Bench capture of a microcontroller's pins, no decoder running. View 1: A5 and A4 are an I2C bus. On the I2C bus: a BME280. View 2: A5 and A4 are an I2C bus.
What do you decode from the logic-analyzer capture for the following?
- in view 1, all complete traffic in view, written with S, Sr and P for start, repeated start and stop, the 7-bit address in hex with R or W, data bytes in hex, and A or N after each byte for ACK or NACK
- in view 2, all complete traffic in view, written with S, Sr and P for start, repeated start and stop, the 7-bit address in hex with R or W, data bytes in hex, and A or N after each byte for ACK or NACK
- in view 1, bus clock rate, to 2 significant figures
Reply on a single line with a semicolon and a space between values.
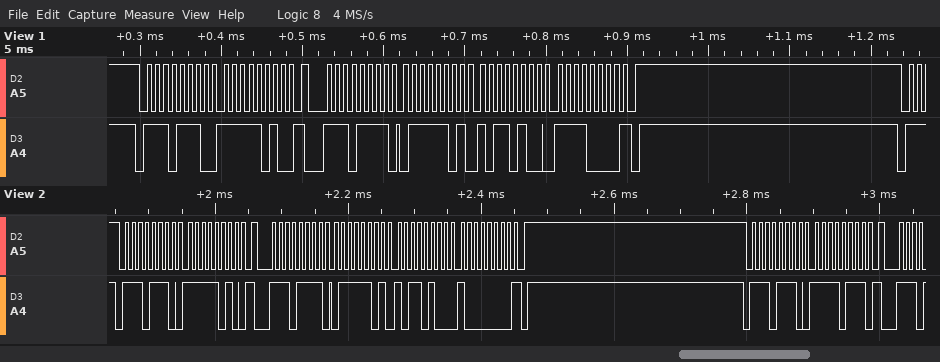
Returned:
S 77W A FA A Sr 77R A 7D A B4 A F0 N P; S 77W A FA A Sr 77R A 7D A B4 A 80 N P S 77W A F7 A; 100 kHz
